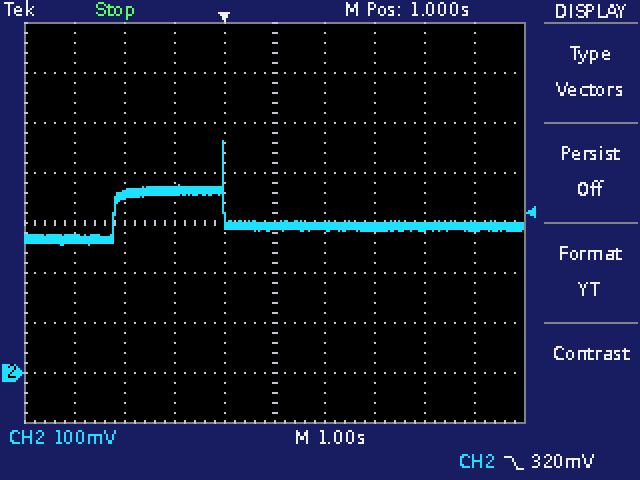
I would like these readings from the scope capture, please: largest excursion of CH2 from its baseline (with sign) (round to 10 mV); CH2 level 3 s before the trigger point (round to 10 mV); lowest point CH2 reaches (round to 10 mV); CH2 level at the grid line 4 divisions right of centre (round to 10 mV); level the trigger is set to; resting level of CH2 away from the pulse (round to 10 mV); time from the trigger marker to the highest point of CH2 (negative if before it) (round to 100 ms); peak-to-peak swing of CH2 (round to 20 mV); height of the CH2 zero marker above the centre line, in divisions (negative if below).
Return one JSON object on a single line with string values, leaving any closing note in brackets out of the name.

{"largest excursion of CH2 from its baseline (with sign)": "+170 mV", "CH2 level 3 s before the trigger point": "270 mV", "lowest point CH2 reaches": "260 mV", "CH2 level at the grid line 4 divisions right of centre": "290 mV", "level the trigger is set to": "320 mV", "resting level of CH2 away from the pulse": "290 mV", "time from the trigger marker to the highest point of CH2 (negative if before it)": "0.0 s", "peak-to-peak swing of CH2": "200 mV", "height of the CH2 zero marker above the centre line, in divisions": "-3.0 div"}
